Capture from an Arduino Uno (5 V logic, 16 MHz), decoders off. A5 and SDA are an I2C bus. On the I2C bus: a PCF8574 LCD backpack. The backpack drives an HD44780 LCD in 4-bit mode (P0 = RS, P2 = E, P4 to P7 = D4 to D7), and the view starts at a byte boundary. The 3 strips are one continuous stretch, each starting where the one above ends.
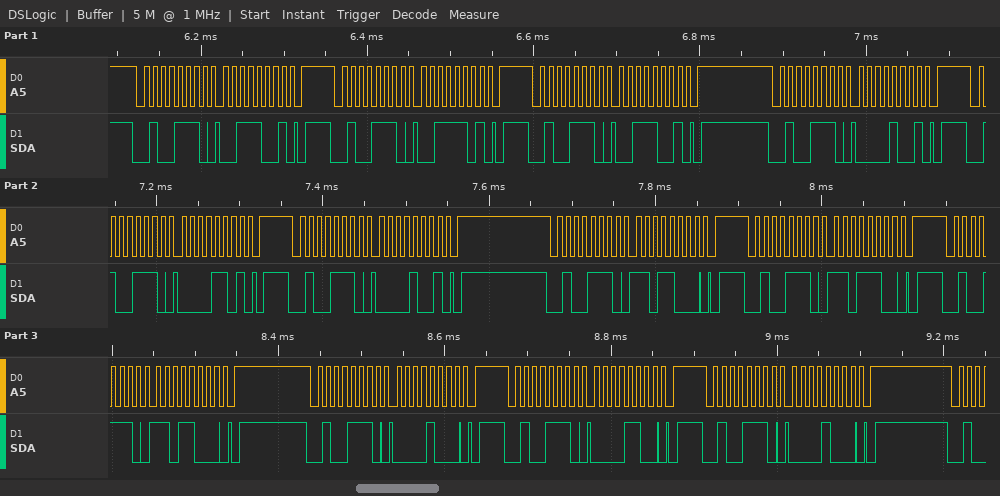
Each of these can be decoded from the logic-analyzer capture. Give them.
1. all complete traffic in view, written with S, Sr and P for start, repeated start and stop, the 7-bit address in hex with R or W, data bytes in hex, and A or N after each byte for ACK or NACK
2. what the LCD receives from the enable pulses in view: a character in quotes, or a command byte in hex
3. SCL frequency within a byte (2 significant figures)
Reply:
S 27W A 39 A P S 27W A 3D A P S 27W A 39 A P S 27W A 09 A P S 27W A 0D A P S 27W A 09 A P S 27W A D8 A P S 27W A DC A P S 27W A D8 A P S 27W A 08 A P S 27W A 0C A P S 27W A 08 A P
'0' 0xD0
100 kHz
